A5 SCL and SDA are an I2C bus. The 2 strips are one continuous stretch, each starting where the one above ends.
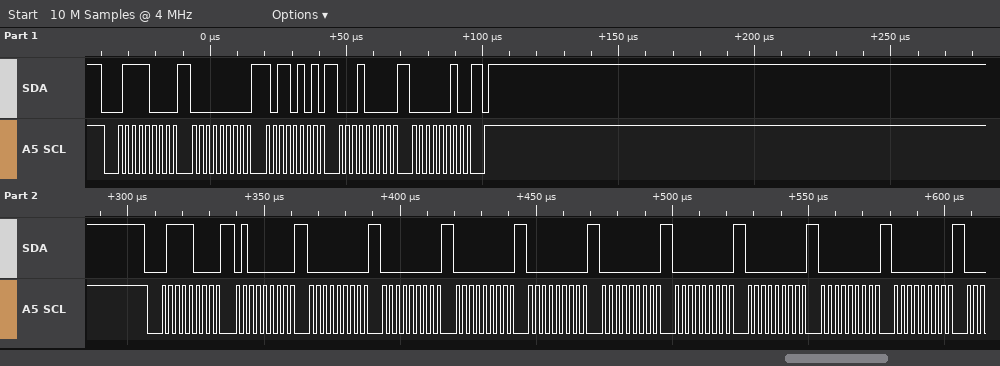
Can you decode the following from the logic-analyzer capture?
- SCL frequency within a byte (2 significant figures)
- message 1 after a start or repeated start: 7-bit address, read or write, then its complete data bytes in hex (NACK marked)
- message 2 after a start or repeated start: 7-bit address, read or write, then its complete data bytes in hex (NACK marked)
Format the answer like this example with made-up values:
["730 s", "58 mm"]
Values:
["400 kHz", "0x3C write: 00 B5 10 02", "0x3C write: 40 00 00 00 00 00 00 00 00 00"]
